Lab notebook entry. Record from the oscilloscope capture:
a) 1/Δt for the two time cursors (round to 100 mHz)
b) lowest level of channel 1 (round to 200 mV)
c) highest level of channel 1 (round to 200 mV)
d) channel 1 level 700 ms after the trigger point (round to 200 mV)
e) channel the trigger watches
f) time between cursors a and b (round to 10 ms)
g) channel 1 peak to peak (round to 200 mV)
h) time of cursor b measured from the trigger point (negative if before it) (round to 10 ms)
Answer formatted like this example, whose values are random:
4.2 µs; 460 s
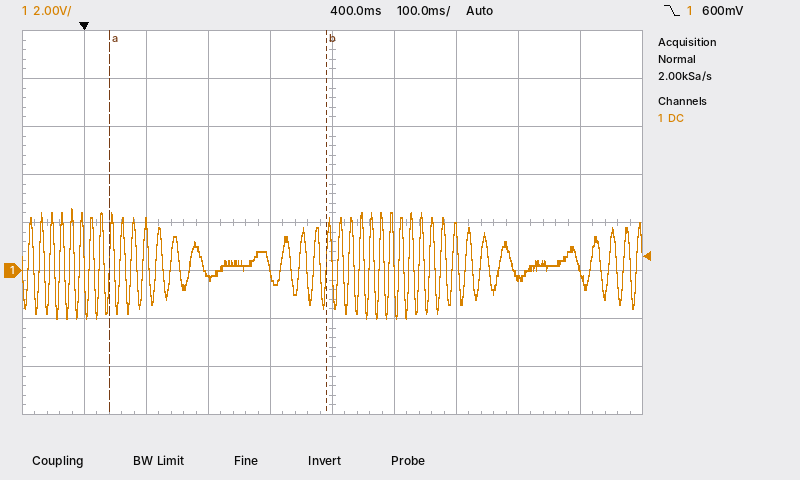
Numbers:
2.9 Hz; -2.0 V; 2.6 V; -200 mV; channel 1; 350 ms; 4.6 V; +390 ms
